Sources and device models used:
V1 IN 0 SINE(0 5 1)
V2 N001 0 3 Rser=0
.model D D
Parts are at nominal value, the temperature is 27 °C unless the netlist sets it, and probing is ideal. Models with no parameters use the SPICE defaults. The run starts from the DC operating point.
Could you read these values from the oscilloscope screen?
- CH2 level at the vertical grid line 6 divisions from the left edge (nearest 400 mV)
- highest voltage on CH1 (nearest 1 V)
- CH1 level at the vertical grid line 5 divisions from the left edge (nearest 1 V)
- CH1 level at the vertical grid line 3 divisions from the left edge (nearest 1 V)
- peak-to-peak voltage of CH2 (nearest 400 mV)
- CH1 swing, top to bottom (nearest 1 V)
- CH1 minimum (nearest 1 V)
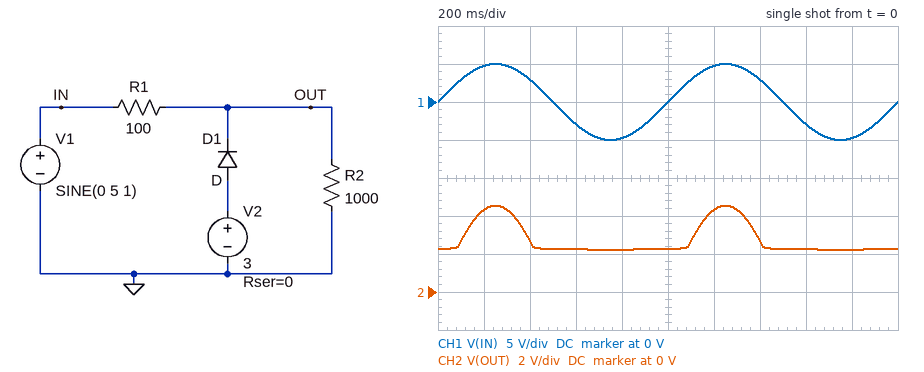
4.4 V
5 V
0 V
-3 V
2.4 V
10 V
-5 V
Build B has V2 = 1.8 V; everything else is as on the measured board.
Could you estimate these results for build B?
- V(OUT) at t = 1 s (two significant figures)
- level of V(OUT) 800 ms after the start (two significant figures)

1.1 V
1.0 V
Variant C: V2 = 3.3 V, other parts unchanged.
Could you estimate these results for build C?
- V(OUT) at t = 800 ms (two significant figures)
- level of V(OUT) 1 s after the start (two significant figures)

2.5 V
2.6 V
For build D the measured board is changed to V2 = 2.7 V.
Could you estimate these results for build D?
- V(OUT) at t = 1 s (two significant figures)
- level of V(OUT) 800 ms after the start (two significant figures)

2.0 V
1.9 V
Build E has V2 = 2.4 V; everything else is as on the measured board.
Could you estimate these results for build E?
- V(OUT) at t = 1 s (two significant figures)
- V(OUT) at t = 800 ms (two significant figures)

1.7 V
1.6 V
